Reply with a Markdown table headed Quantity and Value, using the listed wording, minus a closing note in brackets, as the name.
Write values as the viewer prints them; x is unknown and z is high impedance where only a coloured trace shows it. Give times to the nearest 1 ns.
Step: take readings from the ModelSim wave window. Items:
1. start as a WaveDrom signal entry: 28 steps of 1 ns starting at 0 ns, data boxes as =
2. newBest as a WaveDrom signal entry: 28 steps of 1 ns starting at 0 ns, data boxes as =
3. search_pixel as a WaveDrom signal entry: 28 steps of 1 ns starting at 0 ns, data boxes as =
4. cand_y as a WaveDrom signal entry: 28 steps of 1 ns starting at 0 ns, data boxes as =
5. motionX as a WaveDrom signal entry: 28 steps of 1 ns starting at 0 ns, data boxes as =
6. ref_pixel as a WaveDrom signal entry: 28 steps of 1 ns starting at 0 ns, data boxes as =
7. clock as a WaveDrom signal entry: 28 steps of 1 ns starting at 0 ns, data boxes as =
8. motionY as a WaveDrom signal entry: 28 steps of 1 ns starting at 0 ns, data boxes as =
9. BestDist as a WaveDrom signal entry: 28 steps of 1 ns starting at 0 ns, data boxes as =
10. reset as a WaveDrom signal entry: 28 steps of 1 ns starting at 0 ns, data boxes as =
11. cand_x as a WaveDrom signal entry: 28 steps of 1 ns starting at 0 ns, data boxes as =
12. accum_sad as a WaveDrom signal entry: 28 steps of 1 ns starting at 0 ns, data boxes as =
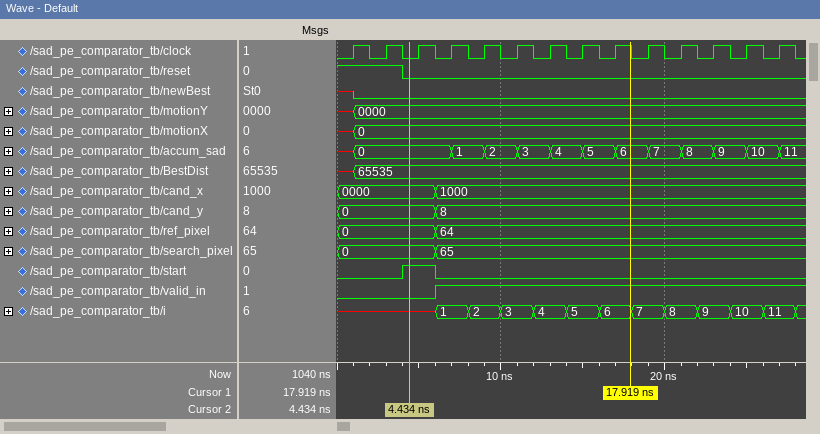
| Quantity | Value |
|---|---|
| start as a WaveDrom signal entry: 28 steps of 1 ns starting at 0 ns, data boxes as = | {name: 'start', wave: '0...1.0.....................'} |
| newBest as a WaveDrom signal entry: 28 steps of 1 ns starting at 0 ns, data boxes as = | {name: 'newBest', wave: 'x0..........................'} |
| search_pixel as a WaveDrom signal entry: 28 steps of 1 ns starting at 0 ns, data boxes as = | {name: 'search_pixel', wave: '=.....=.....................', data: '0 65'} |
| cand_y as a WaveDrom signal entry: 28 steps of 1 ns starting at 0 ns, data boxes as = | {name: 'cand_y', wave: '=.....=.....................', data: '0 8'} |
| motionX as a WaveDrom signal entry: 28 steps of 1 ns starting at 0 ns, data boxes as = | {name: 'motionX', wave: 'x=..........................', data: '0'} |
| ref_pixel as a WaveDrom signal entry: 28 steps of 1 ns starting at 0 ns, data boxes as = | {name: 'ref_pixel', wave: '=.....=.....................', data: '0 64'} |
| clock as a WaveDrom signal entry: 28 steps of 1 ns starting at 0 ns, data boxes as = | {name: 'clock', wave: '0101010101010101010101010101'} |
| motionY as a WaveDrom signal entry: 28 steps of 1 ns starting at 0 ns, data boxes as = | {name: 'motionY', wave: 'x=..........................', data: '0000'} |
| BestDist as a WaveDrom signal entry: 28 steps of 1 ns starting at 0 ns, data boxes as = | {name: 'BestDist', wave: 'x=..........................', data: '65535'} |
| reset as a WaveDrom signal entry: 28 steps of 1 ns starting at 0 ns, data boxes as = | {name: 'reset', wave: '1...0.......................'} |
| cand_x as a WaveDrom signal entry: 28 steps of 1 ns starting at 0 ns, data boxes as = | {name: 'cand_x', wave: '=.....=.....................', data: '0000 1000'} |
| accum_sad as a WaveDrom signal entry: 28 steps of 1 ns starting at 0 ns, data boxes as = | {name: 'accum_sad', wave: 'x=.....=.=.=.=.=.=.=.=.=.=.=', data: '0 1 2 3 4 5 6 7 8 9 10 11'} |
